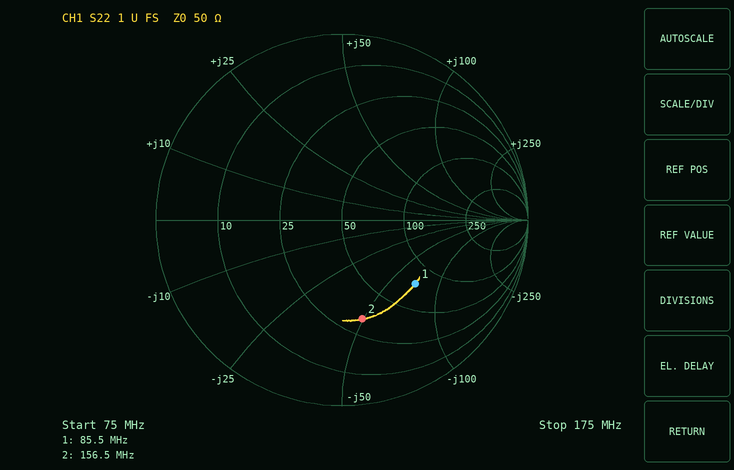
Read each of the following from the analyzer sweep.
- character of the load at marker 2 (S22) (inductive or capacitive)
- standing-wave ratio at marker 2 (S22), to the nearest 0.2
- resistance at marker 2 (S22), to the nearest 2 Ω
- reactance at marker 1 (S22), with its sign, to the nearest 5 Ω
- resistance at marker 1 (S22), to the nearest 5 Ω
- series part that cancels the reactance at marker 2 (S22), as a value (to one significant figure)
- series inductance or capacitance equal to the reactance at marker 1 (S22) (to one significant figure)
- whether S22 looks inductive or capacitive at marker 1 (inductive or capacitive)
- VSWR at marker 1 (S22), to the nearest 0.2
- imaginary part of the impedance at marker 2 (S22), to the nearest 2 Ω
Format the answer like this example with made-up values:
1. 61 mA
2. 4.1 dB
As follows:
1. capacitive
2. 3.4
3. 32 Ω
4. -70 Ω
5. 75 Ω
6. 50 nH
7. 30 pF
8. capacitive
9. 3.2
10. -50 Ω
